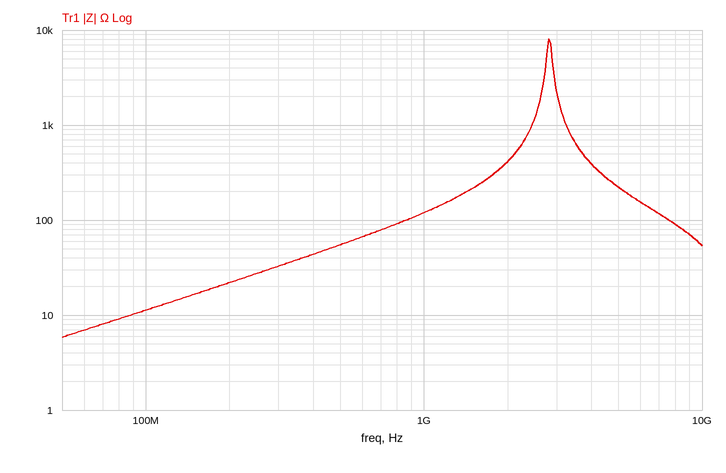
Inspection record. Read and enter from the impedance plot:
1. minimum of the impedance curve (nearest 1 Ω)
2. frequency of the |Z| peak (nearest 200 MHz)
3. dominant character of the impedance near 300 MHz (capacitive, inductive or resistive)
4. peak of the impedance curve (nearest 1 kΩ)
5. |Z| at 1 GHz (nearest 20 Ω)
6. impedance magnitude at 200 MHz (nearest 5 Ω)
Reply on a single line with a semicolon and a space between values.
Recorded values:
6 Ω; 2.8 GHz; inductive; 8 kΩ; 120 Ω; 20 Ω
